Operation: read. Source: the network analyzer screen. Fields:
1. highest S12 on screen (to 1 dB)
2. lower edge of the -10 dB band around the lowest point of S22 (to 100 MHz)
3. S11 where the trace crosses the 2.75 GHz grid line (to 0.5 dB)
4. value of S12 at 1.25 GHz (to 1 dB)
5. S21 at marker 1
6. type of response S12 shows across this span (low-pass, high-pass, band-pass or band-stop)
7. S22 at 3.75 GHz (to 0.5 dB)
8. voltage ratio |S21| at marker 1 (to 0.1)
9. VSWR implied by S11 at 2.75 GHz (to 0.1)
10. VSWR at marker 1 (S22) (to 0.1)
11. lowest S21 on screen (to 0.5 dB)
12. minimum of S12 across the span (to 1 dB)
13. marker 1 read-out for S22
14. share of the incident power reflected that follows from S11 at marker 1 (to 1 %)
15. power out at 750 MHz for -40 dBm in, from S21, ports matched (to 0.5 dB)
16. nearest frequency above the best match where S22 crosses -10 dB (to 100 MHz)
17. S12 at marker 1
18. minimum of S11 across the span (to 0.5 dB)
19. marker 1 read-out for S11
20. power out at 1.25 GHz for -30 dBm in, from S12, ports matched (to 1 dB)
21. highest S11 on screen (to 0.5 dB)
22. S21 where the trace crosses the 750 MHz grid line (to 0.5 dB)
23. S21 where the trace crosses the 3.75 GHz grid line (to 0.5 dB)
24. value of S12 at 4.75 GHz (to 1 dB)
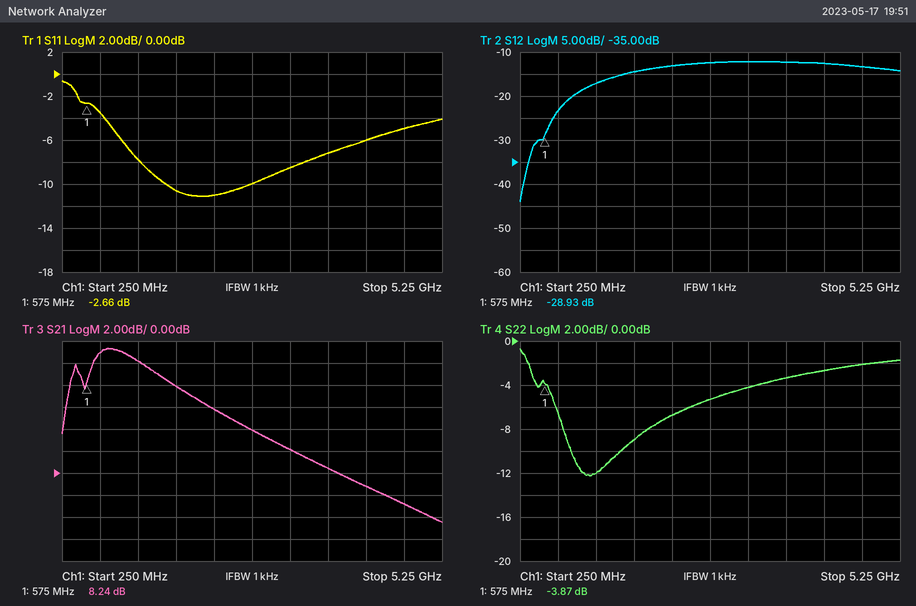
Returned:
-12 dB
900 MHz
-10.0 dB
-17 dB
8.24 dB
high-pass
-3.5 dB
2.6
1.9
4.6
-4.5 dB
-44 dB
-3.87 dB
54 %
-29.0 dBm
1.6 GHz
-28.93 dB
-11.0 dB
-2.66 dB
-47 dBm
-0.5 dB
11.0 dB
0.5 dB
-13 dB
